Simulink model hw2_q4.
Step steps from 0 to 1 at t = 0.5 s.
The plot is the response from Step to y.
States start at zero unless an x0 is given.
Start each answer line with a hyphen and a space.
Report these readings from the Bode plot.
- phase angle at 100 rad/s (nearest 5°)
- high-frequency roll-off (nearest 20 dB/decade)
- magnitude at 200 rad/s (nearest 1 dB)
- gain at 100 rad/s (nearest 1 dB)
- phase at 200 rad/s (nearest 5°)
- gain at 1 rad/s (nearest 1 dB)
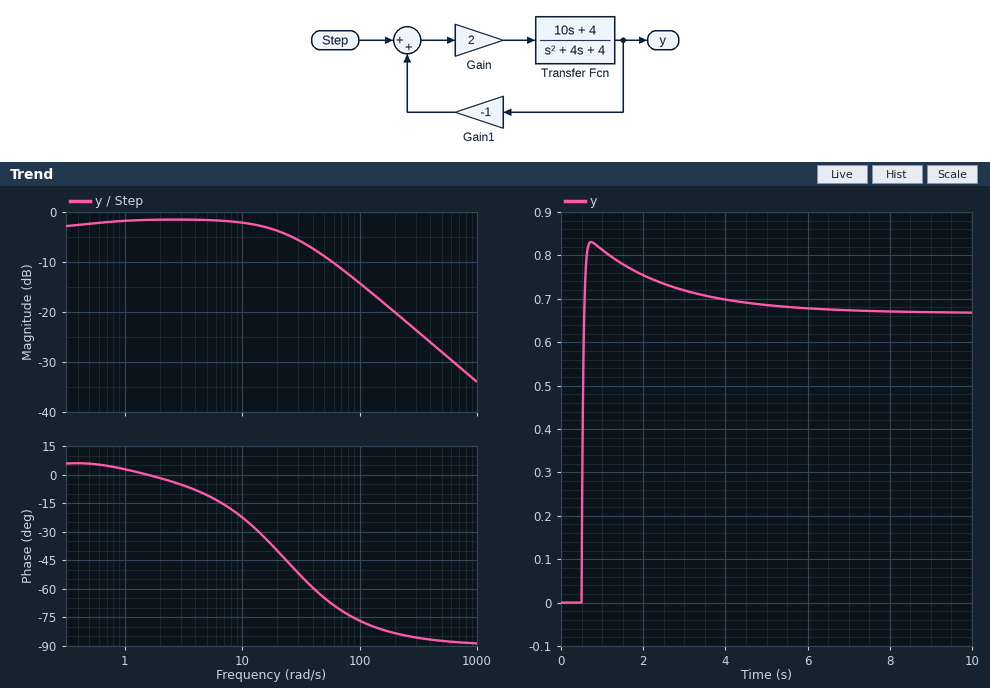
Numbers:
- -75°
- -20 dB/decade
- -20 dB
- -14 dB
- -85°
- -2 dB
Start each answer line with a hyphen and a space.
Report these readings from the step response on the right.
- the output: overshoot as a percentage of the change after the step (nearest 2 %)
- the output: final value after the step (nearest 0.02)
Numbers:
- 24 %
- 0.66
